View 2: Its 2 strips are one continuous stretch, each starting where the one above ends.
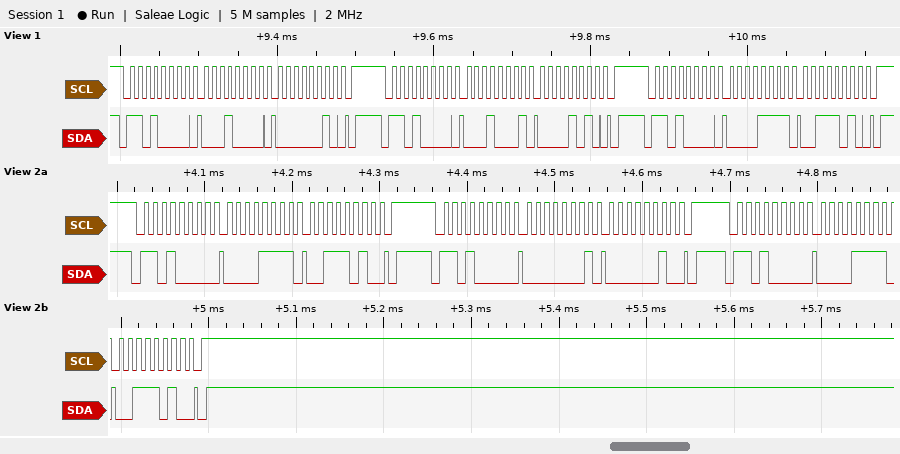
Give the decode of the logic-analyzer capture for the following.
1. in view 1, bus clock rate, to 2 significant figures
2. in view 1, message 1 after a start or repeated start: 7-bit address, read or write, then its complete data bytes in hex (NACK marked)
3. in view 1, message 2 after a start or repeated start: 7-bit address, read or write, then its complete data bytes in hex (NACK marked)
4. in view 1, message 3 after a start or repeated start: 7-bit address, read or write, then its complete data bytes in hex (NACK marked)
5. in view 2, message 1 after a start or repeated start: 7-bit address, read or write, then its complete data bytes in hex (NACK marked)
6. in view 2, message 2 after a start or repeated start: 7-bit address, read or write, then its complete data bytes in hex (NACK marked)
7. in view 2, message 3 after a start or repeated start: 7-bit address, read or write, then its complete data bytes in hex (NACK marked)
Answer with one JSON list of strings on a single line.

["100 kHz", "0x68 write: 10 02", "0x68 write: 11 0A", "0x68 write: 0F 3A", "0x68 write: 0F 3A", "0x68 write: 01 02", "0x68 write: 0F 3A"]
